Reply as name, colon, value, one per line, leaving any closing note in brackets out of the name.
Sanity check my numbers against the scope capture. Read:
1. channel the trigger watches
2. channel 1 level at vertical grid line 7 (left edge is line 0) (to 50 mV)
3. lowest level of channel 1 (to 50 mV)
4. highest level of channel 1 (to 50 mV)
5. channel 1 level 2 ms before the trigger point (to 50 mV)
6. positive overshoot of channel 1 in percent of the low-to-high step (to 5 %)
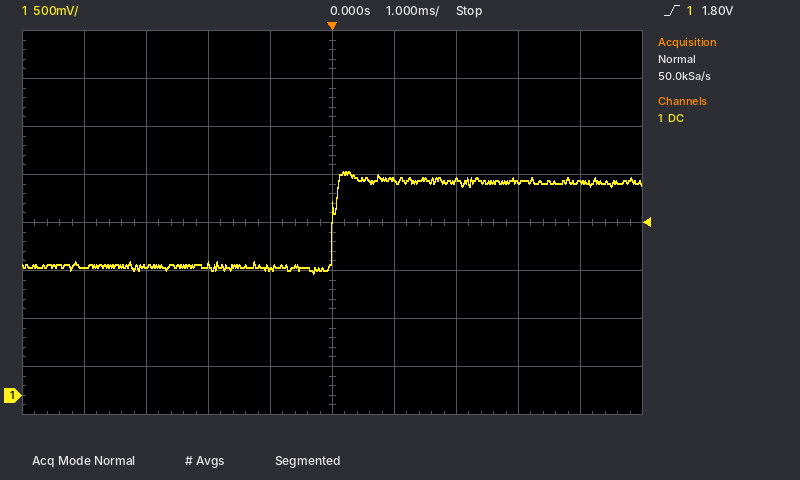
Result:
channel the trigger watches: channel 1
channel 1 level at vertical grid line 7 (left edge is line 0): 2.25 V
lowest level of channel 1: 1.25 V
highest level of channel 1: 2.35 V
channel 1 level 2 ms before the trigger point: 1.35 V
positive overshoot of channel 1 in percent of the low-to-high step: 10 %
